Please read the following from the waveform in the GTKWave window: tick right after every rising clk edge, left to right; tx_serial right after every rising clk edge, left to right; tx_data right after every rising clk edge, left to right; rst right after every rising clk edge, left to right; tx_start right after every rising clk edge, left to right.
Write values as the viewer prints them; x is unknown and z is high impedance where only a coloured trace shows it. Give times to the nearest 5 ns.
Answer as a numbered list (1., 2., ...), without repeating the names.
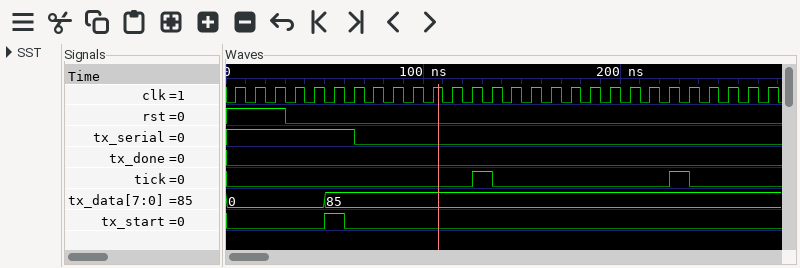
1. 0 0 0 0 0 0 0 0 0 0 0 0 1 0 0 0 0 0 0 0 0 0 1 0 0 0 0 0
2. 1 1 1 1 1 1 0 0 0 0 0 0 0 0 0 0 0 0 0 0 0 0 0 0 0 0 0 0
3. 0, 0, 0, 0, 0, 85, 85, 85, 85, 85, 85, 85, 85, 85, 85, 85, 85, 85, 85, 85, 85, 85, 85, 85, 85, 85, 85, 85
4. 1 1 1 0 0 0 0 0 0 0 0 0 0 0 0 0 0 0 0 0 0 0 0 0 0 0 0 0
5. 0 0 0 0 0 1 0 0 0 0 0 0 0 0 0 0 0 0 0 0 0 0 0 0 0 0 0 0
